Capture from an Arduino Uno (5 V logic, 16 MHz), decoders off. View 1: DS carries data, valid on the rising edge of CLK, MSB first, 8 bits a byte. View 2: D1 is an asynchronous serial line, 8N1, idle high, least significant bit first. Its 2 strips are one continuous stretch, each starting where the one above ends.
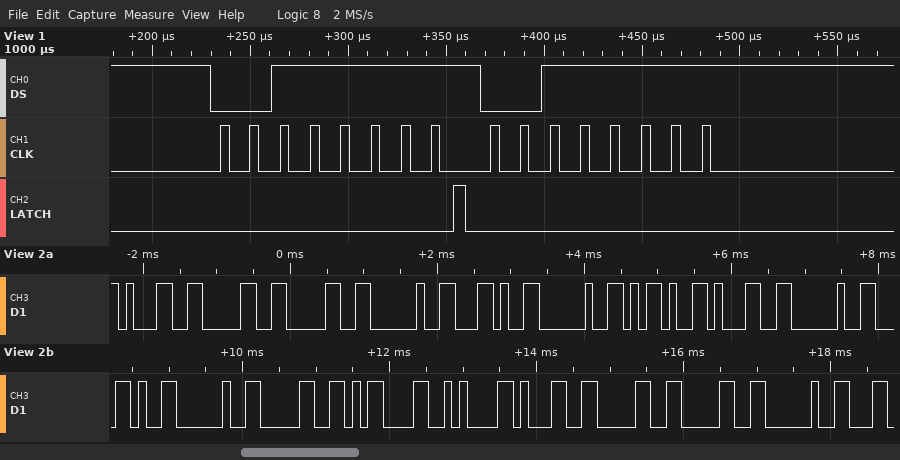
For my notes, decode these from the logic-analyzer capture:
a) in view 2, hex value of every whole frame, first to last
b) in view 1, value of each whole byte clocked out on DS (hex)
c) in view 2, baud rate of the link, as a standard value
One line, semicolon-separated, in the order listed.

31 30 30 20 2C 20 2D 31 20 2C 20 30 0D 0A 31 30 30 20; 0x3F 0x3F; 9600 baud
